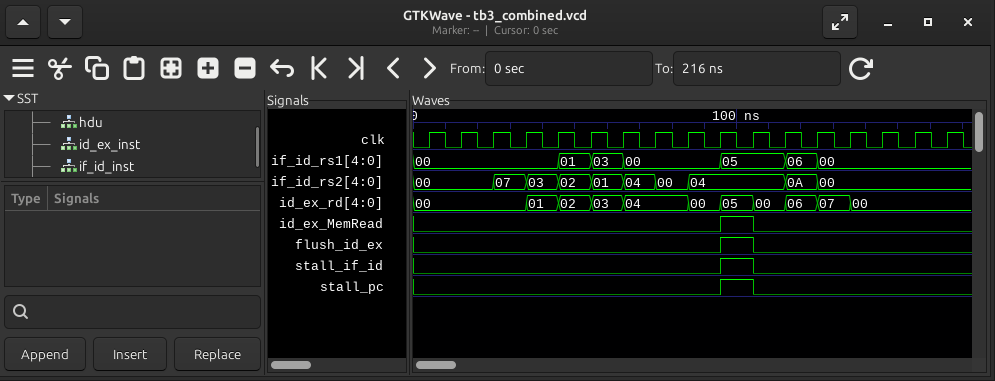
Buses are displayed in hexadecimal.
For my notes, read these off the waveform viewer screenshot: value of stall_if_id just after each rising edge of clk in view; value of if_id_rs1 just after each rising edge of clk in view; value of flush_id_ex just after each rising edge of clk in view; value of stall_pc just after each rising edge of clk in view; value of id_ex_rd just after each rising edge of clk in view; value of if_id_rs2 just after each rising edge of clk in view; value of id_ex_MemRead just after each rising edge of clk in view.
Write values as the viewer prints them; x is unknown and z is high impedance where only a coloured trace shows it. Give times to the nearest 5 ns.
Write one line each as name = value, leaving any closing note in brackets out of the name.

value of stall_if_id just after each rising edge of clk in view = 0 0 0 0 0 0 0 0 0 1 0 0 0 0 0 0 0
value of if_id_rs1 just after each rising edge of clk in view = 00, 00, 00, 00, 01, 03, 00, 00, 00, 05, 05, 06, 00, 00, 00, 00, 00
value of flush_id_ex just after each rising edge of clk in view = 0 0 0 0 0 0 0 0 0 1 0 0 0 0 0 0 0
value of stall_pc just after each rising edge of clk in view = 0 0 0 0 0 0 0 0 0 1 0 0 0 0 0 0 0
value of id_ex_rd just after each rising edge of clk in view = 00, 00, 00, 01, 02, 03, 04, 04, 00, 05, 00, 06, 07, 00, 00, 00, 00
value of if_id_rs2 just after each rising edge of clk in view = 00, 00, 07, 03, 02, 01, 04, 00, 04, 04, 04, 0A, 00, 00, 00, 00, 00
value of id_ex_MemRead just after each rising edge of clk in view = 0 0 0 0 0 0 0 0 0 1 0 0 0 0 0 0 0
